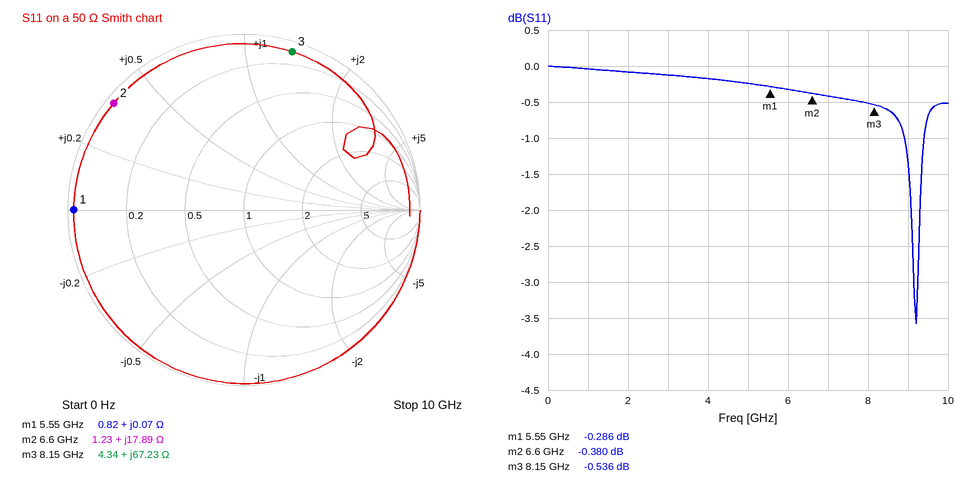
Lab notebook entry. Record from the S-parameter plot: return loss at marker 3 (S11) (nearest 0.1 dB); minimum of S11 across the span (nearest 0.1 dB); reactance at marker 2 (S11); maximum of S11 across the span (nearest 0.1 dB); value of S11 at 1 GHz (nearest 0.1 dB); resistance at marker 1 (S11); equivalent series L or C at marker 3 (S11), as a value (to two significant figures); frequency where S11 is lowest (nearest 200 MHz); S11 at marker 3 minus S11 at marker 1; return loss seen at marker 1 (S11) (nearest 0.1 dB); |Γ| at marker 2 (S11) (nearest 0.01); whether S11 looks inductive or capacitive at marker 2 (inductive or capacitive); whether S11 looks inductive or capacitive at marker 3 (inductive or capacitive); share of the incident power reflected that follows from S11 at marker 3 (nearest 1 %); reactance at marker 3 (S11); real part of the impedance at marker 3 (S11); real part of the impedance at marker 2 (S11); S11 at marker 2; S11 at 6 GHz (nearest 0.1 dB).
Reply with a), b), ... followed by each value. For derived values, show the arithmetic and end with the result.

a) 0.5 dB
b) -3.6 dB
c) +17.89 Ω
d) 0.0 dB
e) 0.0 dB
f) 0.82 Ω
g) L = 67.23 Ω/(2π × 8.15 GHz) ≈ 1.3 nH
h) 9.2 GHz
i) -0.536 − (-0.286) = -0.250 dB
j) 0.3 dB
k) 0.96
l) inductive
m) inductive
n) 10^(-0.536/10) ≈ 88 %
o) +67.23 Ω
p) 4.34 Ω
q) 1.23 Ω
r) -0.380 dB
s) -0.3 dB
